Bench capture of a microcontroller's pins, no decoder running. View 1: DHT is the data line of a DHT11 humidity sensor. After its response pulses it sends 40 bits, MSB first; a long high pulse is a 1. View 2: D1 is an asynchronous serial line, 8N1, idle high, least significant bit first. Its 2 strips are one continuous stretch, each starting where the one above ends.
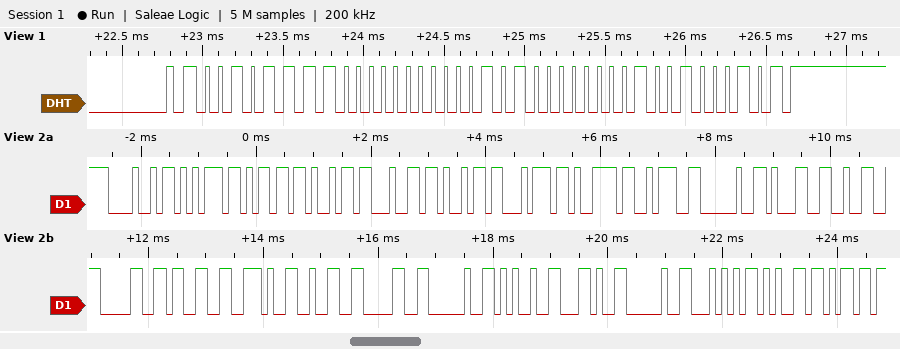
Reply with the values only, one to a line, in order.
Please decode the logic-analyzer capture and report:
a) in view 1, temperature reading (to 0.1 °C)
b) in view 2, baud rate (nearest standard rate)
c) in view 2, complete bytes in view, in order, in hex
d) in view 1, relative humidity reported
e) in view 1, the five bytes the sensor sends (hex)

20.2 °C
9600 baud
48 75 6D 69 64 69 74 79 3A 20 31 32 30 33 2E 32 30 20 25 2C 20 54 65 6D
47 %
2F 00 14 02 45
